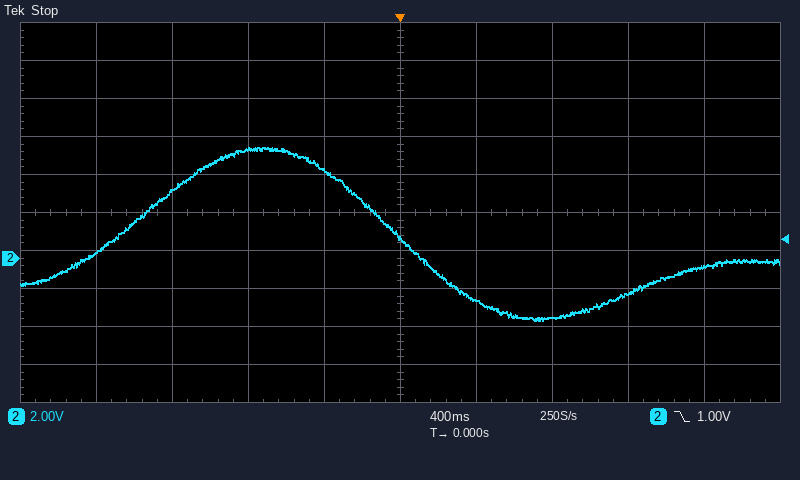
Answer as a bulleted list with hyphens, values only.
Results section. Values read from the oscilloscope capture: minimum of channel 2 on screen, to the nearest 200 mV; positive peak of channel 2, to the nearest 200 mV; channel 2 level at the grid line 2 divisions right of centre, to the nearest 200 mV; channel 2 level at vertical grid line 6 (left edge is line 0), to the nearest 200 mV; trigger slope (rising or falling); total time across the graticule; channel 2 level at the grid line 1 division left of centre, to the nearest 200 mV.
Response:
- -3.2 V
- 5.8 V
- -3.2 V
- -2.2 V
- falling
- 4 s
- 4.6 V
